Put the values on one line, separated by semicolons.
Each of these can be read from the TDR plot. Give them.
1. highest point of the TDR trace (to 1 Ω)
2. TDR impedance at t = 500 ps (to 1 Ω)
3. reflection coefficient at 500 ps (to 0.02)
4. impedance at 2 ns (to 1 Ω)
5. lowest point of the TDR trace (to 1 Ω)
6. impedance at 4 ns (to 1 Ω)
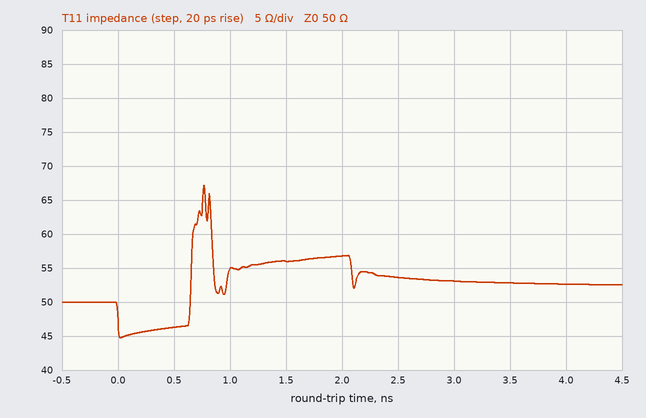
67 Ω; 46 Ω; -0.04; 57 Ω; 45 Ω; 53 Ω
